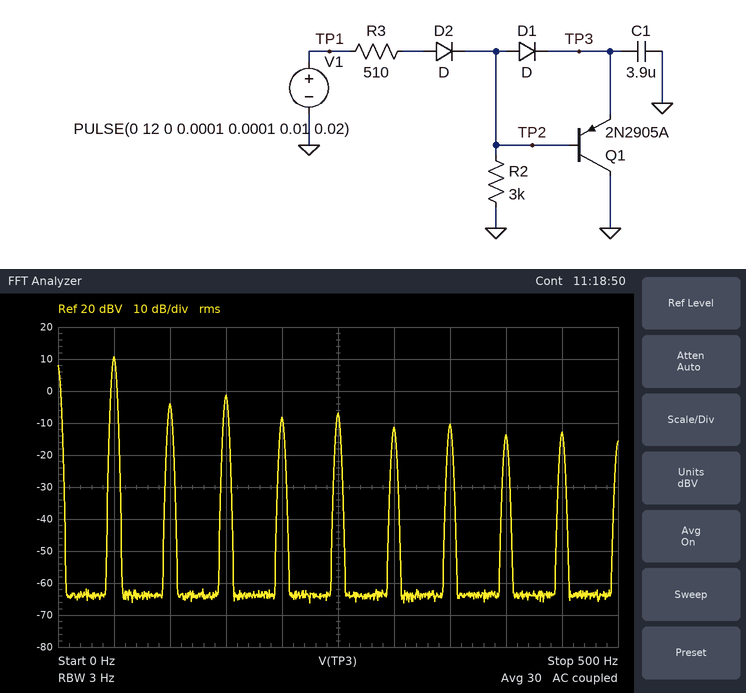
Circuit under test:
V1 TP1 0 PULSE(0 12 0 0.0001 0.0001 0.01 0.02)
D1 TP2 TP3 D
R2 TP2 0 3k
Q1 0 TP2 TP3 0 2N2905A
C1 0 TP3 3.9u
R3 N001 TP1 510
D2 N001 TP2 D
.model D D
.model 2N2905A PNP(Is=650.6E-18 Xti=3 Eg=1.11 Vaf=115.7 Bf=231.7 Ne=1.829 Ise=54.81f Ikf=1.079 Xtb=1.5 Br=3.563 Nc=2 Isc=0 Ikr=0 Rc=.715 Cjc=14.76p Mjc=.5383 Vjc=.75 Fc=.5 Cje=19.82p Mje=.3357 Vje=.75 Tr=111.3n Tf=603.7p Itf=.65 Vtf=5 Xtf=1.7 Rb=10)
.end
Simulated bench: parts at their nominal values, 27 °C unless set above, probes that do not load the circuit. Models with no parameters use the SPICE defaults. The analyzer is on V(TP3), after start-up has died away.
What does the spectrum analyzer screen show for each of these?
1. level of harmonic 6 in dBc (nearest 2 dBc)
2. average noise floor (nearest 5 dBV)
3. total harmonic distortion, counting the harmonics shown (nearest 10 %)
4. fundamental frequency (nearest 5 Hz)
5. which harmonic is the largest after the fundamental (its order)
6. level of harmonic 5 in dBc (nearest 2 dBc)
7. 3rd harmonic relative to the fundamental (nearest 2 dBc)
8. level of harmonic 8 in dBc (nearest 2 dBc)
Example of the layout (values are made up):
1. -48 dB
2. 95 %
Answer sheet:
1. -22 dBc
2. -65 dBV
3. 40 %
4. 50 Hz
5. 3
6. -18 dBc
7. -12 dBc
8. -24 dBc
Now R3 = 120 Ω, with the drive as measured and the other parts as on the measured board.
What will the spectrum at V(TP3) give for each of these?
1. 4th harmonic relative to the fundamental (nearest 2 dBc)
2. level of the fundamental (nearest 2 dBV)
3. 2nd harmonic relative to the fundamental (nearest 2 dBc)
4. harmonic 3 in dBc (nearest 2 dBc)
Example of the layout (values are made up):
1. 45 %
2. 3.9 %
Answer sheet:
1. -26 dBc
2. 12 dBV
3. -26 dBc
4. -10 dBc
